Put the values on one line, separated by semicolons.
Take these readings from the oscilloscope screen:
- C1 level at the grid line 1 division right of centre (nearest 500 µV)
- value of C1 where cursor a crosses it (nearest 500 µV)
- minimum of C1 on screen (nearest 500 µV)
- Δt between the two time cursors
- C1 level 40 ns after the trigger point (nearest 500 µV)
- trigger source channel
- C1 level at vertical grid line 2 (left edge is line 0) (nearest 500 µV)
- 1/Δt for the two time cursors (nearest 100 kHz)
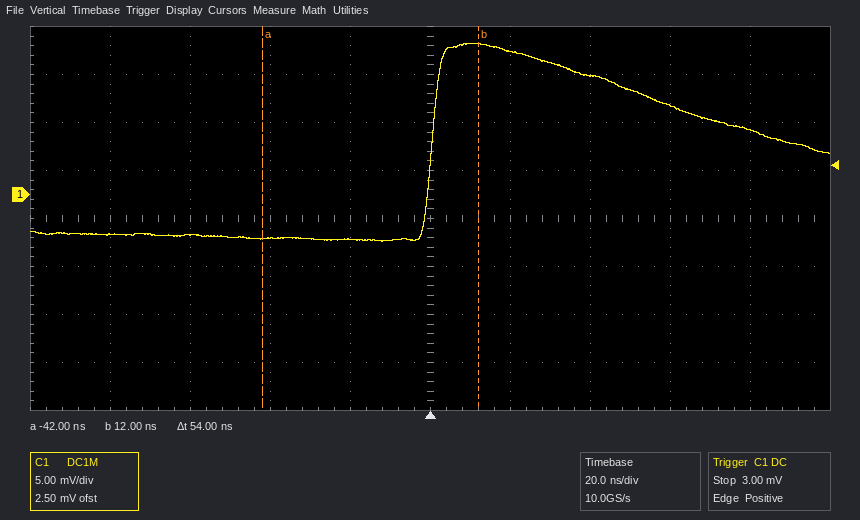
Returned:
15.0 mV; -4.5 mV; -5.0 mV; 54 ns; 12.5 mV; C1; -4.0 mV; 18.5 MHz
